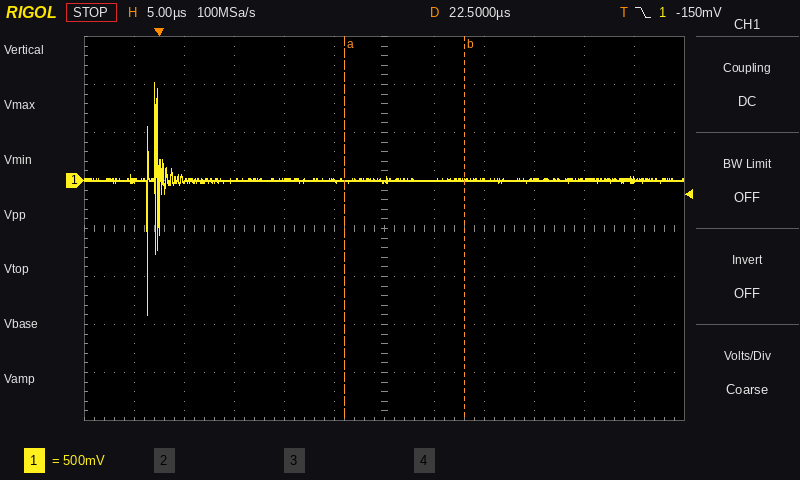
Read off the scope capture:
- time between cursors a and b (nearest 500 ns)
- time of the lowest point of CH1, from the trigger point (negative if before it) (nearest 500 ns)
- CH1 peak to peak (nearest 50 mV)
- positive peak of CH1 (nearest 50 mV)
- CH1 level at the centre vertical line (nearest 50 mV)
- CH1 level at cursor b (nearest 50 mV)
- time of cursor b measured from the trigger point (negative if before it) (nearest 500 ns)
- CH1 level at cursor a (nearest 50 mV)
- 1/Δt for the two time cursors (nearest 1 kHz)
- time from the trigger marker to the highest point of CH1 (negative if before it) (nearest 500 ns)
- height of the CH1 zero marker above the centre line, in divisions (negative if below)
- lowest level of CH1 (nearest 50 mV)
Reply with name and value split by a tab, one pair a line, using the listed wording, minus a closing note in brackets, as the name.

time between cursors a and b	12.0 µs
time of the lowest point of CH1, from the trigger point (negative if before it)	-1.0 µs
CH1 peak to peak	2.40 V
positive peak of CH1	1.00 V
CH1 level at the centre vertical line	0 mV
CH1 level at cursor b	0 mV
time of cursor b measured from the trigger point (negative if before it)	+30.5 µs
CH1 level at cursor a	0 mV
1/Δt for the two time cursors	83 kHz
time from the trigger marker to the highest point of CH1 (negative if before it)	-500 ns
height of the CH1 zero marker above the centre line, in divisions	+1.0 div
lowest level of CH1	-1.40 V
